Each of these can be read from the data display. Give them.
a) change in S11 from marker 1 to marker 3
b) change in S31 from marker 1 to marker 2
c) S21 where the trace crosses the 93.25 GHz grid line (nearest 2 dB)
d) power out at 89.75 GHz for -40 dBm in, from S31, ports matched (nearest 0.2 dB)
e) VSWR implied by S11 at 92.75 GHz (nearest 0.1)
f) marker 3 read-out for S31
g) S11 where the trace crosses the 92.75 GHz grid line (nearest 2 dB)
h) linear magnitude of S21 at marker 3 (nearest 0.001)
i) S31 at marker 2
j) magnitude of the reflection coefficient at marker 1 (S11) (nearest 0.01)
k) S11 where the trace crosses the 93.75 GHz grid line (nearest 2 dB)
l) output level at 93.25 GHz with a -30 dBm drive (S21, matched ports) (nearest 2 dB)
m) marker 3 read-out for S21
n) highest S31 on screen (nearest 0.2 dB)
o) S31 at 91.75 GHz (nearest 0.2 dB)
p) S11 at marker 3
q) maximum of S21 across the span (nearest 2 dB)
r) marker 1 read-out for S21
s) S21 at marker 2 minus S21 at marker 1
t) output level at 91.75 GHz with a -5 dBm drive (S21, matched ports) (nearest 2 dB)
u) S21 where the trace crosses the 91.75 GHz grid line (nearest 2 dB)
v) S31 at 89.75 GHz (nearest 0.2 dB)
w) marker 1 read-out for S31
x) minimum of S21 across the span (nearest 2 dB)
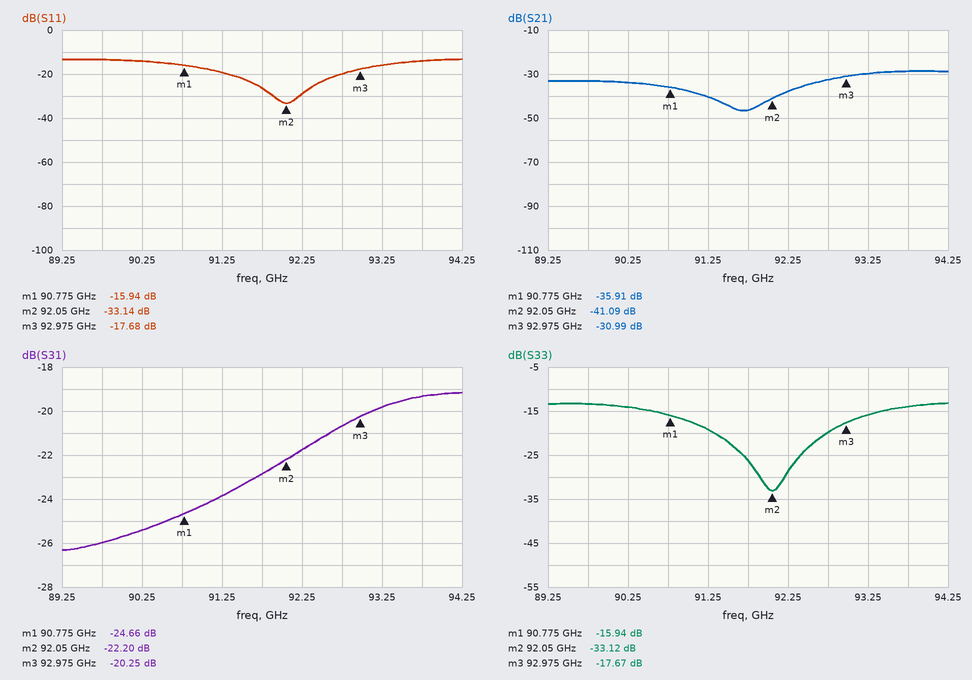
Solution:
-1.74 dB
2.46 dB
-30 dB
-66.0 dBm
1.2
-20.25 dB
-20 dB
0.028
-22.20 dB
0.16
-14 dB
-60 dBm
-30.99 dB
-19.2 dB
-22.8 dB
-17.68 dB
-28 dB
-35.91 dB
-5.18 dB
-52 dBm
-46 dB
-26.0 dB
-24.66 dB
-46 dB
